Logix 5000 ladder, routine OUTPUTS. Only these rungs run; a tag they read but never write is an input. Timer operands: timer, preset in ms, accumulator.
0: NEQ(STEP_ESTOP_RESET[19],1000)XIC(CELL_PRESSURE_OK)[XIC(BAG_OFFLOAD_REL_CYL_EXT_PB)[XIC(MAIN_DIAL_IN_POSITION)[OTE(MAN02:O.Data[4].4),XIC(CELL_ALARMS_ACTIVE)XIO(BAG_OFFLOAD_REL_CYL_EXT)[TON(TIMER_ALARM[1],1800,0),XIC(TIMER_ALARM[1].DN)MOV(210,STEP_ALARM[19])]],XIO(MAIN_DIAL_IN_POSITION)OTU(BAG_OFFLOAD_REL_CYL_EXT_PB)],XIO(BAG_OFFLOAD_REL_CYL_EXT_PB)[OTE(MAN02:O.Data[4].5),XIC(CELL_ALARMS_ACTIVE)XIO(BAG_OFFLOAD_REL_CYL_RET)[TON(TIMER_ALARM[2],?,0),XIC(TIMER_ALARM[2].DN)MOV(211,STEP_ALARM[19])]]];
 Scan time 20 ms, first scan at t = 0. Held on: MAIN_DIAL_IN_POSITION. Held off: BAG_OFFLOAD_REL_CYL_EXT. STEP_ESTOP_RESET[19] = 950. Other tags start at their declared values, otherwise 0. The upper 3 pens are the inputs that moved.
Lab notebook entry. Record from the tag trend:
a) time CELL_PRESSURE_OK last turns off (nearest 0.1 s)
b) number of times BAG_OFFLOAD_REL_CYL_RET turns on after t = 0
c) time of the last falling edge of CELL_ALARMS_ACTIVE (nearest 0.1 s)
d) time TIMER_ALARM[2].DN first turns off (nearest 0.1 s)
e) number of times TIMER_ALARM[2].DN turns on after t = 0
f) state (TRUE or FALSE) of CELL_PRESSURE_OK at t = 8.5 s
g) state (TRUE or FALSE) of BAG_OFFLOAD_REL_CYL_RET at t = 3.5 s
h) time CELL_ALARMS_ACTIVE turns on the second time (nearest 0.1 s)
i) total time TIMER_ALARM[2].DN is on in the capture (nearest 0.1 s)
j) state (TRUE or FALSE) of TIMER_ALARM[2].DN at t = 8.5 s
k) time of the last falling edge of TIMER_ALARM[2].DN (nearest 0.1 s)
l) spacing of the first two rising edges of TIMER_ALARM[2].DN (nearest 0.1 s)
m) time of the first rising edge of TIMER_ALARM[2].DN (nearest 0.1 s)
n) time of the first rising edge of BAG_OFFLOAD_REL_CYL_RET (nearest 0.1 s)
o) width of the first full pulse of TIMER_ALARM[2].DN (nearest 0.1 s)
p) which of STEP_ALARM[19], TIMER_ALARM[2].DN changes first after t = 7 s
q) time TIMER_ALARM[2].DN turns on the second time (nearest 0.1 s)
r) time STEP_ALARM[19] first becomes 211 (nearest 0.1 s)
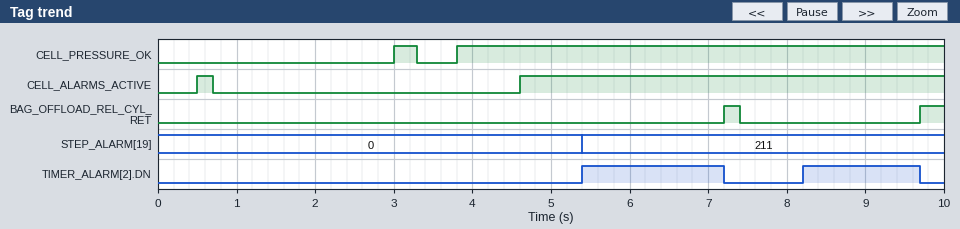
3.3 s
2
0.7 s
7.2 s
2
TRUE
FALSE
4.6 s
3.3 s
TRUE
9.7 s
2.8 s
5.4 s
7.2 s
1.8 s
TIMER_ALARM[2].DN
8.2 s
5.4 s
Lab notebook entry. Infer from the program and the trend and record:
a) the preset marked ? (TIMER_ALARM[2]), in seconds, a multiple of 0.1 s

0.8 s
